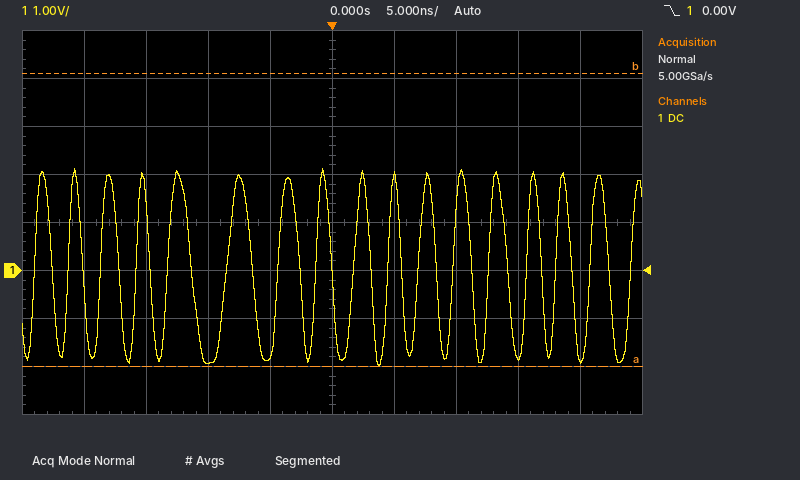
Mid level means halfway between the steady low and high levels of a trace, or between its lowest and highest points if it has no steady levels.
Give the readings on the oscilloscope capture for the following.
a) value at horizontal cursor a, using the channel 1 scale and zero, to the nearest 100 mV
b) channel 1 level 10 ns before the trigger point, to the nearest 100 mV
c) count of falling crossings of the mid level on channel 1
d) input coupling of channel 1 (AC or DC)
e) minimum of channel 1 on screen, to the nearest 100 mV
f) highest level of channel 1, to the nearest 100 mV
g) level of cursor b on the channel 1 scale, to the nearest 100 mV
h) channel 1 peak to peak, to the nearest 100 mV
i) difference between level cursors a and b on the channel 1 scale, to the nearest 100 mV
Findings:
-2.0 V
-1.9 V
16
DC
-2.0 V
2.1 V
4.1 V
4.1 V
6.1 V
